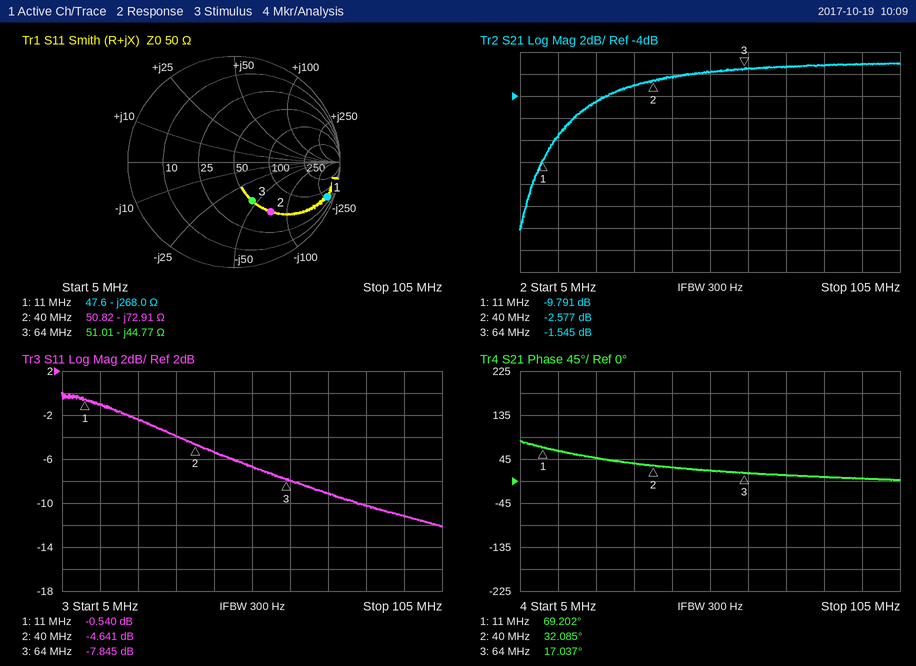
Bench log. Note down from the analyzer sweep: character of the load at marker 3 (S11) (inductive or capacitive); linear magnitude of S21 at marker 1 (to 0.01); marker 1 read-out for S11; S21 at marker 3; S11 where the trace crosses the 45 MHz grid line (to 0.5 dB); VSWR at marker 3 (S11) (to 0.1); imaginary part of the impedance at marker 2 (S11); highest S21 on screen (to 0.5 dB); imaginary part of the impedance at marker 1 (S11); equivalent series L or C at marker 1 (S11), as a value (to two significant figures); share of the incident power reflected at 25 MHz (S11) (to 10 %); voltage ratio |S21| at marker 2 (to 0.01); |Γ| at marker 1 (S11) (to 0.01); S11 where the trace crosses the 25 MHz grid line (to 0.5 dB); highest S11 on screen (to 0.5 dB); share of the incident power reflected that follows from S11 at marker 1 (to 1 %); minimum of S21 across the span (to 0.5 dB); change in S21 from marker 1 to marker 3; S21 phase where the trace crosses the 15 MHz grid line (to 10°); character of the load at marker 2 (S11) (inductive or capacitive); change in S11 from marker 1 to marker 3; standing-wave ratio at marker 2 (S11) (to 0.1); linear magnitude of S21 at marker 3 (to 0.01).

capacitive
0.32
-0.540 dB
-1.545 dB
-5.5 dB
2.4
-72.91 Ω
-1.0 dB
-268.0 Ω
54 pF
60 %
0.74
0.94
-2.5 dB
0.0 dB
88 %
-16.0 dB
8.246 dB
60°
capacitive
-7.305 dB
3.8
0.84
